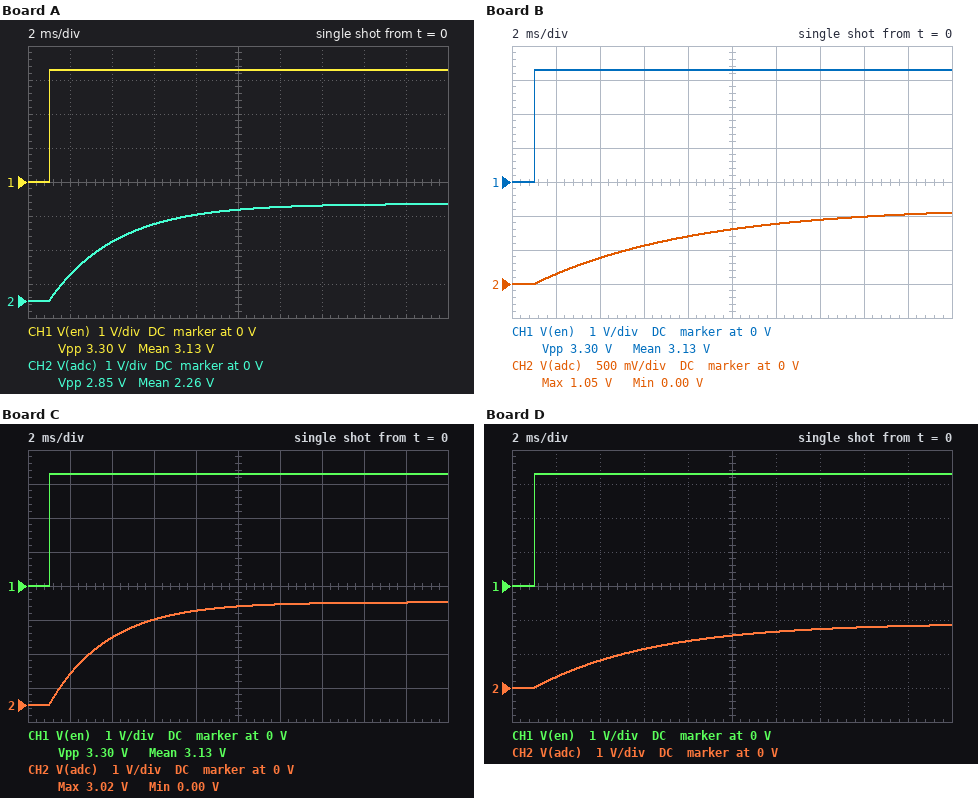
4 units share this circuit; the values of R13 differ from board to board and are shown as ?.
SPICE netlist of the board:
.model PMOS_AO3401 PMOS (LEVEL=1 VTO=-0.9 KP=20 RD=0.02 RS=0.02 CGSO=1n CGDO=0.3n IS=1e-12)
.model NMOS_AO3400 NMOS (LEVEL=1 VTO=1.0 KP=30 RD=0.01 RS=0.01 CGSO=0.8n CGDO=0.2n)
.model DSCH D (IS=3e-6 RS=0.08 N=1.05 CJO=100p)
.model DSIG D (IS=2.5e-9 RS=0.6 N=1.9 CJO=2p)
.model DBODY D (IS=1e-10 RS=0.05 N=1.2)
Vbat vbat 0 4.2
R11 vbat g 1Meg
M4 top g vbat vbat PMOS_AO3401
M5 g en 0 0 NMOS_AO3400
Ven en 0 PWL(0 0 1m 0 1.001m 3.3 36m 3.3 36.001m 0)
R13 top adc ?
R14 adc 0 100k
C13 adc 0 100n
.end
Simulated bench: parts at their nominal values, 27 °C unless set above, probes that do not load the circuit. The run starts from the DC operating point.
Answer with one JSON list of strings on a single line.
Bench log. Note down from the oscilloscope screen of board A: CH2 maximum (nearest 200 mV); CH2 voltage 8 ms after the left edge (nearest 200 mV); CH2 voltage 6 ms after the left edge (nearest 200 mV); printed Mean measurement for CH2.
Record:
["2.8 V", "2.6 V", "2.2 V", "2.26 V"]
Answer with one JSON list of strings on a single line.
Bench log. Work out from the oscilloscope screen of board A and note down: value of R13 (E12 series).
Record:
["47 kΩ"]
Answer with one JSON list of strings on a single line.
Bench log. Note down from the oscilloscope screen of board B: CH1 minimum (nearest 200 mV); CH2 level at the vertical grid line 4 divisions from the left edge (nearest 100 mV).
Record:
["0 V", "700 mV"]
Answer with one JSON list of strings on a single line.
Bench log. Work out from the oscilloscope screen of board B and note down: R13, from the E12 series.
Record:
["270 kΩ"]
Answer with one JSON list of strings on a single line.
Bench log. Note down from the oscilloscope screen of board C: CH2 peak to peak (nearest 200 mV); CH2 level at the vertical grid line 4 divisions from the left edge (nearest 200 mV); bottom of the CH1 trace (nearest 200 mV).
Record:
["3.0 V", "2.8 V", "0 V"]
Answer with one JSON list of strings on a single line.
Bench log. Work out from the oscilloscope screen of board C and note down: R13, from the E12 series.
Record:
["39 kΩ"]
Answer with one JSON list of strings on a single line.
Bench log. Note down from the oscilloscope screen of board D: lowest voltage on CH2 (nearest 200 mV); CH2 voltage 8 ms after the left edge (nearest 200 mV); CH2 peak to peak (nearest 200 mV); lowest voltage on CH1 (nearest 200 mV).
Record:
["0 V", "1.4 V", "1.8 V", "0 V"]
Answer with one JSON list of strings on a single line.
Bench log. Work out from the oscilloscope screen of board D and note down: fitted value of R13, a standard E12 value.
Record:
["120 kΩ"]
